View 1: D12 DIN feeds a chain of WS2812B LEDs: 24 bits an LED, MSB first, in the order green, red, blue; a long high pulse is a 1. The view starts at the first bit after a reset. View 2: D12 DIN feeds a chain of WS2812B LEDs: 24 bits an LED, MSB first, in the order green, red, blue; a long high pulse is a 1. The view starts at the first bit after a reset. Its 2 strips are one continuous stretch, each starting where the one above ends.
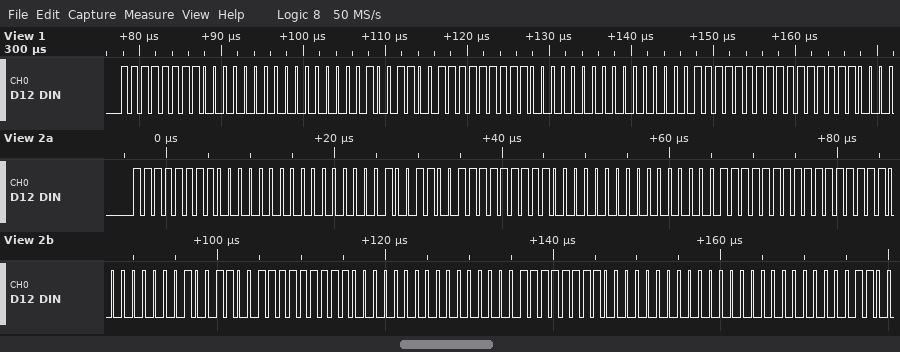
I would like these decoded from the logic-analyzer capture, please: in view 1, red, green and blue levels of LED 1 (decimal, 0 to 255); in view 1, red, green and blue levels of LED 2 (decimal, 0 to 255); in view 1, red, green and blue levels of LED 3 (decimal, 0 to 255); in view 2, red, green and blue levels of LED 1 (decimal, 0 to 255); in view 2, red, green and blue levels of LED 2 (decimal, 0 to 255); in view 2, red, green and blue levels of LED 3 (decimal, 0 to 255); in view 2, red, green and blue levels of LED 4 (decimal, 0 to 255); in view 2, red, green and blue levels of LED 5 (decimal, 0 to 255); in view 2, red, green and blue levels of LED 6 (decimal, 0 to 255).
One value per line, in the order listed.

0, 255, 0
255, 153, 0
255, 0, 255
0, 255, 0
255, 153, 0
255, 0, 255
153, 0, 255
0, 0, 255
0, 0, 0
